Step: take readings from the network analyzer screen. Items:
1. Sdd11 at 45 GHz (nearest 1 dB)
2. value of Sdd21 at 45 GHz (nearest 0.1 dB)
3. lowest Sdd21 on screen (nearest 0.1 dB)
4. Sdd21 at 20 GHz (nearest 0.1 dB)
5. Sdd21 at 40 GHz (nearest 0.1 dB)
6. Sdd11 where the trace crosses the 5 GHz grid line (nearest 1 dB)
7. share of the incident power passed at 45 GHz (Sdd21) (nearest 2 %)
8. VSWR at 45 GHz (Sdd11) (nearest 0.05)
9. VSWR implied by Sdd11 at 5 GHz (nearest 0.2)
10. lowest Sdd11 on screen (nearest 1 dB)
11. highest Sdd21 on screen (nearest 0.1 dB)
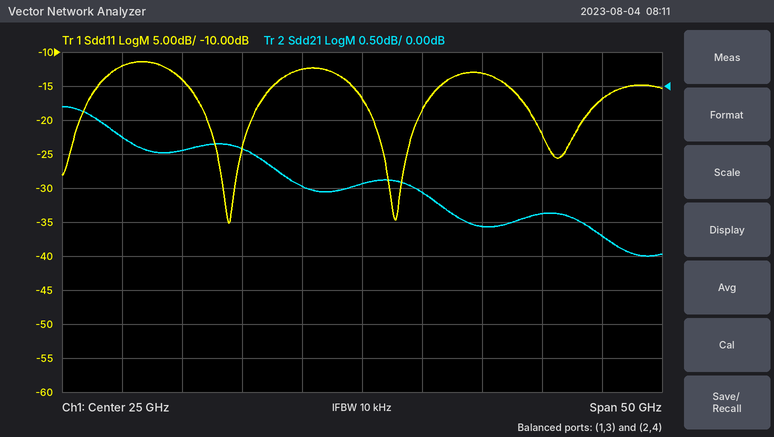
-17 dB
-2.2 dB
-2.5 dB
-1.5 dB
-1.9 dB
-12 dB
60 %
1.35
1.6
-35 dB
-0.3 dB
